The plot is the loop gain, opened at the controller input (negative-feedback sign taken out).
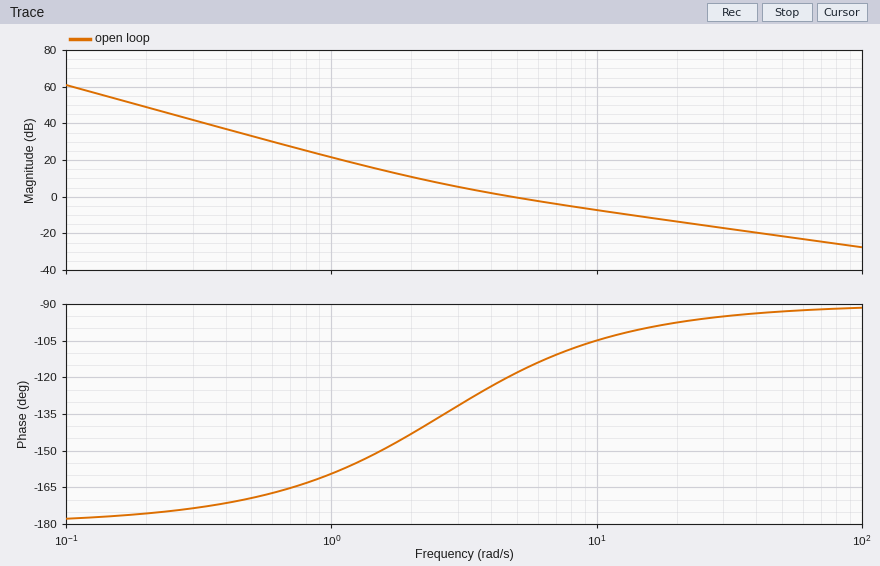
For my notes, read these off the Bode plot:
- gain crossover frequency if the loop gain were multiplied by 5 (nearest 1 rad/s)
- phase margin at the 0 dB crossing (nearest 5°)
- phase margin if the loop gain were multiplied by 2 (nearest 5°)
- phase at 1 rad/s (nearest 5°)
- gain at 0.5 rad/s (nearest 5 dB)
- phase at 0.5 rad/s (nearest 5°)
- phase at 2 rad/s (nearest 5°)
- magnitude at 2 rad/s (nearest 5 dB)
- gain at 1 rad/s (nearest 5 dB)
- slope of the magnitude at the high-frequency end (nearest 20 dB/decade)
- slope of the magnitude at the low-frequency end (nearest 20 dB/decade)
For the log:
21 rad/s
60°
75°
-160°
35 dB
-170°
-145°
10 dB
20 dB
-20 dB/decade
-40 dB/decade
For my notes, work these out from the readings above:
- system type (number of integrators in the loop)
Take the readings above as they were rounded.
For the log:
2
